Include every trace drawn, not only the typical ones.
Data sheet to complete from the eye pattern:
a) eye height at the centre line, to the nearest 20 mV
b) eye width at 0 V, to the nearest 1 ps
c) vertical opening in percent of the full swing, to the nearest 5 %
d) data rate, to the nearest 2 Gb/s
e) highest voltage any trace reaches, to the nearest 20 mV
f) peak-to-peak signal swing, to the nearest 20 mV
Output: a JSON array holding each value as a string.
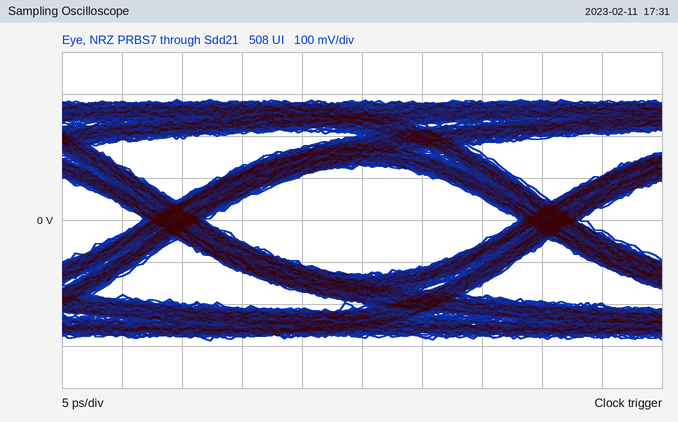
["260 mV", "26 ps", "45 %", "32 Gb/s", "280 mV", "580 mV"]
